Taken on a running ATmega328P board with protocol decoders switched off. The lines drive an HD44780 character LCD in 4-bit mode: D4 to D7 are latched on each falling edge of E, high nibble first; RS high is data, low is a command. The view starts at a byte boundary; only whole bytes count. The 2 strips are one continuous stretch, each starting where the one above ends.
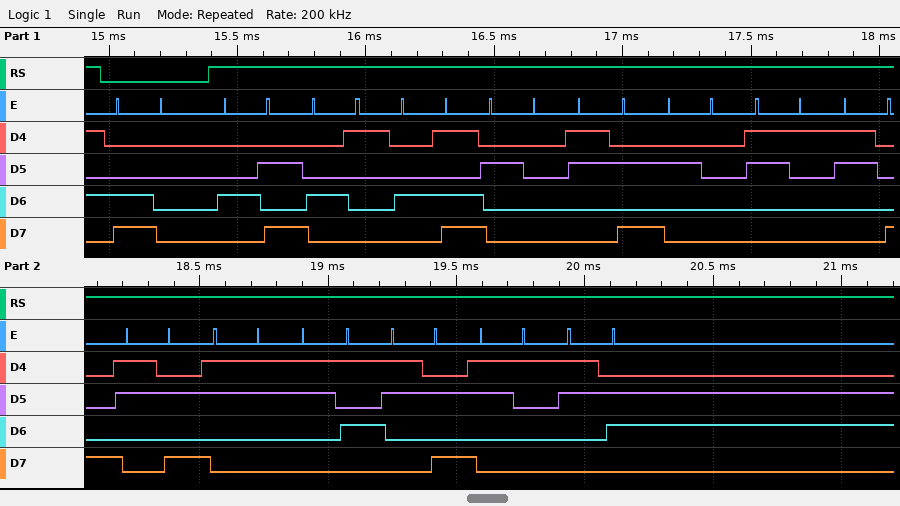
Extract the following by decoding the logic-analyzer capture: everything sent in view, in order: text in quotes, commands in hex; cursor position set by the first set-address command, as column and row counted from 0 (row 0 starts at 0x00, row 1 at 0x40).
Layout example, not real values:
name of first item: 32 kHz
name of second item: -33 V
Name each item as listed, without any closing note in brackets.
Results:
everything sent in view, in order: text in quotes, commands in hex: 0xC0 "JAM : 18:35:16"
cursor position set by the first set-address command, as column and row counted from 0: column 0, row 1
